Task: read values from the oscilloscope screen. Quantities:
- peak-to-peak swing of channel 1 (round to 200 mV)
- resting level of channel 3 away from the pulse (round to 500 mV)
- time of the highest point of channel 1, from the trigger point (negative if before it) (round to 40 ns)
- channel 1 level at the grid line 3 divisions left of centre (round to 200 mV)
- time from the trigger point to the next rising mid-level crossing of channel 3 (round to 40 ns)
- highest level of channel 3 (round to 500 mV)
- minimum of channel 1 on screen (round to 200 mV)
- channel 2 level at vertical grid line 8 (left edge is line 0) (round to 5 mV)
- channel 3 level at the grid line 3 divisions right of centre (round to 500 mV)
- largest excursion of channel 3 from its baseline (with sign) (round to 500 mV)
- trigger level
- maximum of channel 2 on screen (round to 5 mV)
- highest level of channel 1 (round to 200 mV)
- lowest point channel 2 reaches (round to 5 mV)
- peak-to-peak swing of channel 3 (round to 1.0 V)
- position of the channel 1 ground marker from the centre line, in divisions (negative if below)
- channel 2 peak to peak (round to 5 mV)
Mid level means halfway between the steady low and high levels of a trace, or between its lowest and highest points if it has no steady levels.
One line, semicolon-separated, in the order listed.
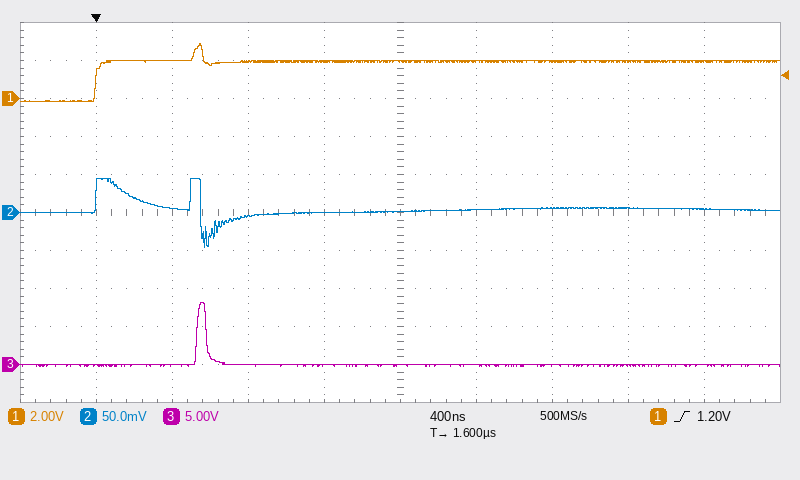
3.0 V; 0.0 V; +560 ns; 2.0 V; 520 ns; 8.0 V; -200 mV; 5 mV; 0.0 V; +8.0 V; 1.20 V; 45 mV; 2.8 V; -45 mV; 8.0 V; +3.0 div; 90 mV
